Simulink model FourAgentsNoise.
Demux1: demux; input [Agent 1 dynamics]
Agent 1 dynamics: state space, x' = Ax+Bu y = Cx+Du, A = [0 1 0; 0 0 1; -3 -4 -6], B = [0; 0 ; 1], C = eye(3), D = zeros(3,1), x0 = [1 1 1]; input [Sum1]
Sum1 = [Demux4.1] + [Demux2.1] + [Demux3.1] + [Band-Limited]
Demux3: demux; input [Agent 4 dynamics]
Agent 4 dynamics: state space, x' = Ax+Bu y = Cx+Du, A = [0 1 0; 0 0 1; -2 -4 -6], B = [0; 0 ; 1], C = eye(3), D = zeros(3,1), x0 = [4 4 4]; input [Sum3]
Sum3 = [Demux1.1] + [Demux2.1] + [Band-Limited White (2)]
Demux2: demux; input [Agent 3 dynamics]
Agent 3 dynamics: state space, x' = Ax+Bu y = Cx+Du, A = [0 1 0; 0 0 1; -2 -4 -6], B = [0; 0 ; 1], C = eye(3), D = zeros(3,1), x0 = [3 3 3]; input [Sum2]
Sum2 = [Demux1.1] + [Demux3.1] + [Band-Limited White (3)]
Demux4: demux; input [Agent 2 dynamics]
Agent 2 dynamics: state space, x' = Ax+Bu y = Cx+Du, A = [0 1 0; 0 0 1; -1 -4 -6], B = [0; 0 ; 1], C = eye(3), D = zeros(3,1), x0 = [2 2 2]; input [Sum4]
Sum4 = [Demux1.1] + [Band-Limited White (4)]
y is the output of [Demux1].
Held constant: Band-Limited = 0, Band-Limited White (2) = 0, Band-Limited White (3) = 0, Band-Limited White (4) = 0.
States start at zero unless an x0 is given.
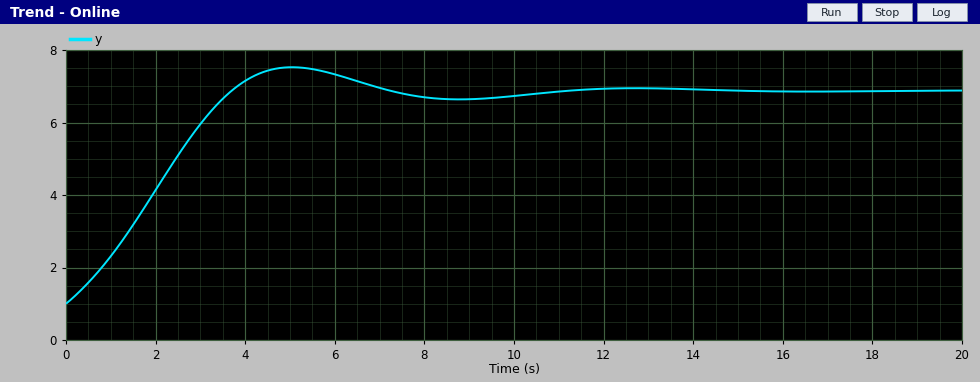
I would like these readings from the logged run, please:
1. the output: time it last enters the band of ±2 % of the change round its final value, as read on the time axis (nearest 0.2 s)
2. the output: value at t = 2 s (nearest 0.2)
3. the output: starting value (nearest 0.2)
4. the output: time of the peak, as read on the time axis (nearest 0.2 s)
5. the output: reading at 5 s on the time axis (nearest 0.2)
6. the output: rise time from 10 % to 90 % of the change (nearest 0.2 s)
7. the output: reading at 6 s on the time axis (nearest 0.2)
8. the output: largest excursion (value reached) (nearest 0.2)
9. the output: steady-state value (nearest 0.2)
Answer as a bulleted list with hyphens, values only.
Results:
- 10.2 s
- 4.2
- 1.0
- 5.0 s
- 7.6
- 2.8 s
- 7.4
- 7.6
- 6.8
